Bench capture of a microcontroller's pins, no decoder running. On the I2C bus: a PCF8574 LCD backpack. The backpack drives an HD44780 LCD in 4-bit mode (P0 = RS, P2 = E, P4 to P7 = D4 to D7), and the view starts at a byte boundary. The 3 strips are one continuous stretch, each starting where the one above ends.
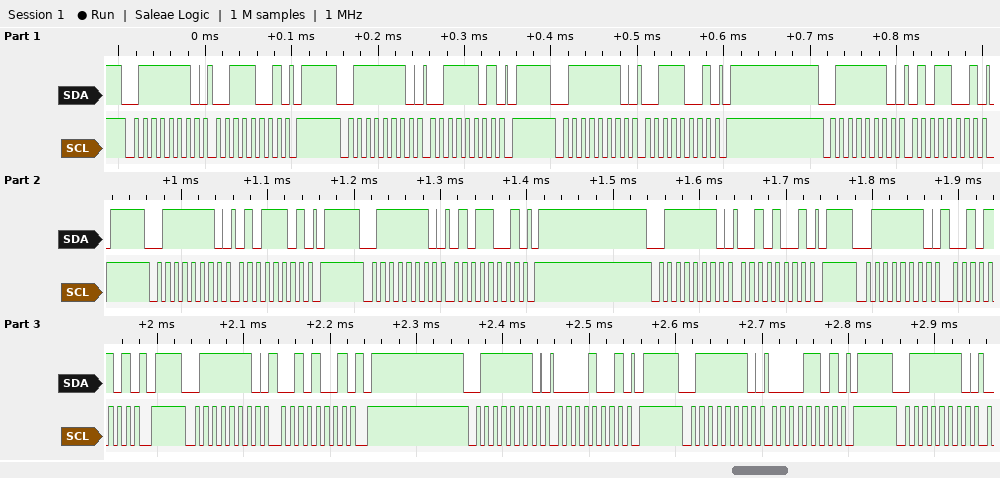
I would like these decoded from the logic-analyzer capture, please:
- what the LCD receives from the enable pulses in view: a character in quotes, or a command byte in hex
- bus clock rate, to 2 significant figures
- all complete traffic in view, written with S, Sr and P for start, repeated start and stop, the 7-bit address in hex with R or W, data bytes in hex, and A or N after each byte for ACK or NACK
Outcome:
'5'
100 kHz
S 3FW A 39 A P S 3FW A 3D A P S 3FW A 39 A P S 3FW A 59 A P S 3FW A 5D A P S 3FW A 59 A P S 3FW A 29 A P S 3FW A 2D A P S 3FW A 29 A P S 3FW A 09 A P S 3FW A 0D A P S 3FW A
